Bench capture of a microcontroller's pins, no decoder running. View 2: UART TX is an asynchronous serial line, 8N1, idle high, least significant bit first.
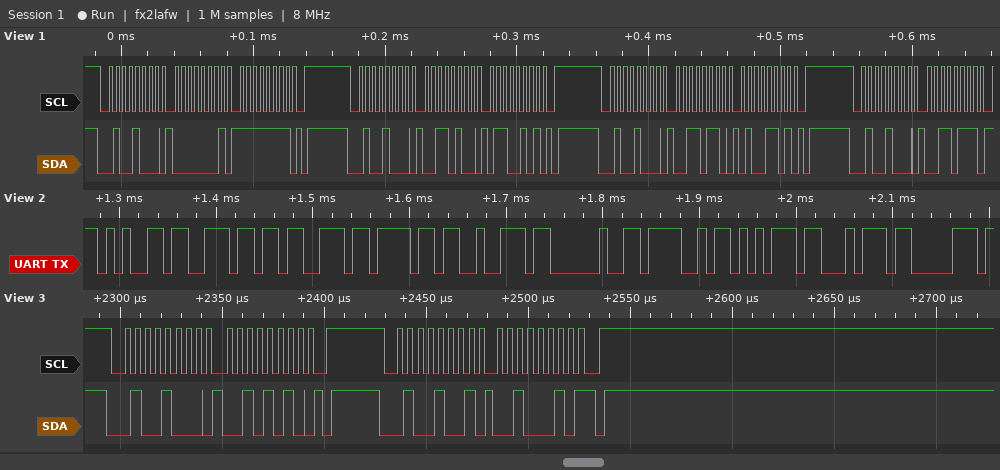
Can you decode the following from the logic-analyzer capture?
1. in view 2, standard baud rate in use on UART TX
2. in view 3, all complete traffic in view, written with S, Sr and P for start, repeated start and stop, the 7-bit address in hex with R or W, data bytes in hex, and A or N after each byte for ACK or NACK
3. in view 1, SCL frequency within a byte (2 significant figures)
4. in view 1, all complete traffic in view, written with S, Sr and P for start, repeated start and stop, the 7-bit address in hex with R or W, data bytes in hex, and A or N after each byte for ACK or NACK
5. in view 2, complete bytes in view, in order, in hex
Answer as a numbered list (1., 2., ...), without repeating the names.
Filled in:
1. 115200 baud
2. S 24W A 2A A P S 24R A 22 N P
3. 200 kHz
4. S 24W A 01 A FF A P S 24W A 34 A 65 A P S 24W A 36 A 4D A P S 24W A 37 A
5. 65 6E 73 6F 72 20 4F 75 74 70
